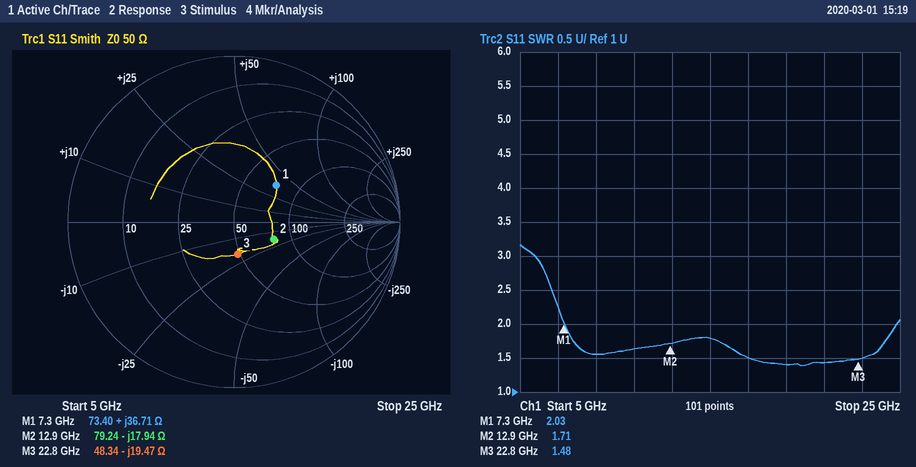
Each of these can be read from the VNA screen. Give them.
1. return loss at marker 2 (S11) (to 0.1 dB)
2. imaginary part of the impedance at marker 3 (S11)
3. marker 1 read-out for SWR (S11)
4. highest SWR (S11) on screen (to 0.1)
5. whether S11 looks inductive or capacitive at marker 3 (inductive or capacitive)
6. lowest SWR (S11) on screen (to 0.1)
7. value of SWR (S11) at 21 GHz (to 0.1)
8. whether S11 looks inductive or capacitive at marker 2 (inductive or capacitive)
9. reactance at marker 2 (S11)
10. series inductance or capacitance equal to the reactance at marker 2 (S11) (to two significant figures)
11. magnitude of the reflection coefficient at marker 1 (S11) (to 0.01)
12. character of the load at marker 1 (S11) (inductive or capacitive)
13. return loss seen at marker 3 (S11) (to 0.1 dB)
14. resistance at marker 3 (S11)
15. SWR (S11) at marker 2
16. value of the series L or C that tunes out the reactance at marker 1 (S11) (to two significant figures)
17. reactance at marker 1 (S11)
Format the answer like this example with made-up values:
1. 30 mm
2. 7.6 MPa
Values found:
1. 11.6 dB
2. -19.47 Ω
3. 2.03
4. 3.2
5. capacitive
6. 1.4
7. 1.4
8. capacitive
9. -17.94 Ω
10. 690 fF
11. 0.34
12. inductive
13. 14.2 dB
14. 48.34 Ω
15. 1.71
16. 590 fF
17. +36.71 Ω
